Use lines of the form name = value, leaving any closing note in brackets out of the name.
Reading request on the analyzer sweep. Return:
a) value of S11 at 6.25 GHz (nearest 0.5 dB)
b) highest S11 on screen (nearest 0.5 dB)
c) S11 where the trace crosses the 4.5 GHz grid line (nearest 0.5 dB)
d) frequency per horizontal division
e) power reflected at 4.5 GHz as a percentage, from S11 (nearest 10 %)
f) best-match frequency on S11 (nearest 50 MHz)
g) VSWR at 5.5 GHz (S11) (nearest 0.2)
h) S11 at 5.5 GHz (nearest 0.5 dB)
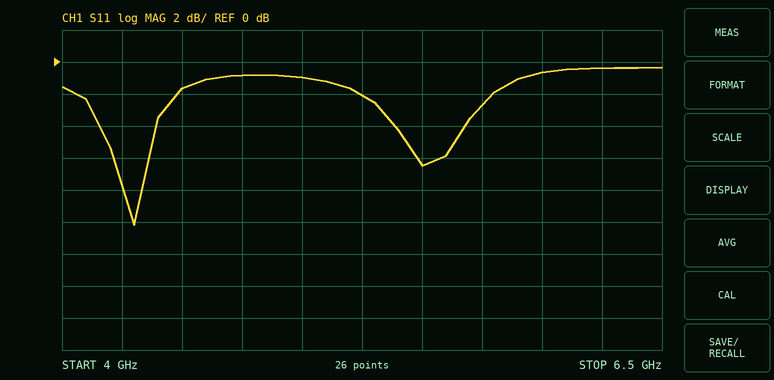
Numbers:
value of S11 at 6.25 GHz = -0.5 dB
highest S11 on screen = -0.5 dB
S11 where the trace crosses the 4.5 GHz grid line = -1.5 dB
frequency per horizontal division = 250 MHz
power reflected at 4.5 GHz as a percentage, from S11 = 70 %
best-match frequency on S11 = 4.30 GHz
VSWR at 5.5 GHz (S11) = 2.8
S11 at 5.5 GHz = -6.5 dB
